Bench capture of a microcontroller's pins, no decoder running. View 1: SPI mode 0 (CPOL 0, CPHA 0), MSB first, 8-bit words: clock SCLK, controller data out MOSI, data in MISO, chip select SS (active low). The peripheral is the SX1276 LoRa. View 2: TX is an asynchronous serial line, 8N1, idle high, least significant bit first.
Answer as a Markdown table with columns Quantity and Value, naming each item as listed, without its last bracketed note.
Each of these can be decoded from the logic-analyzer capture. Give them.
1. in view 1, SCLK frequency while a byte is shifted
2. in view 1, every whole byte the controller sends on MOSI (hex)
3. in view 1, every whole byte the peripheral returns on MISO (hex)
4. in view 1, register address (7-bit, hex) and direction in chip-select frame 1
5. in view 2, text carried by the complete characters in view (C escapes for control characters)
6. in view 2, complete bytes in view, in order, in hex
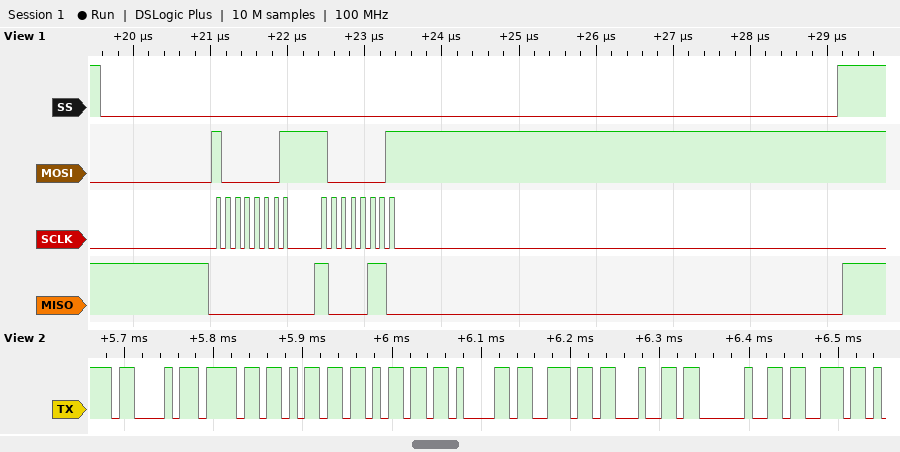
| Quantity | Value |
|---|---|
| in view 1, SCLK frequency while a byte is shifted | 8 MHz |
| in view 1, every whole byte the controller sends on MOSI | 81 81 |
| in view 1, every whole byte the peripheral returns on MISO | 00 86 |
| in view 1, register address (7-bit, hex) and direction in chip-select frame 1 | 0x01 write |
| in view 2, text carried by the complete characters in view | "Command s" |
| in view 2, complete bytes in view, in order, in hex | 43 6F 6D 6D 61 6E 64 20 73 |
